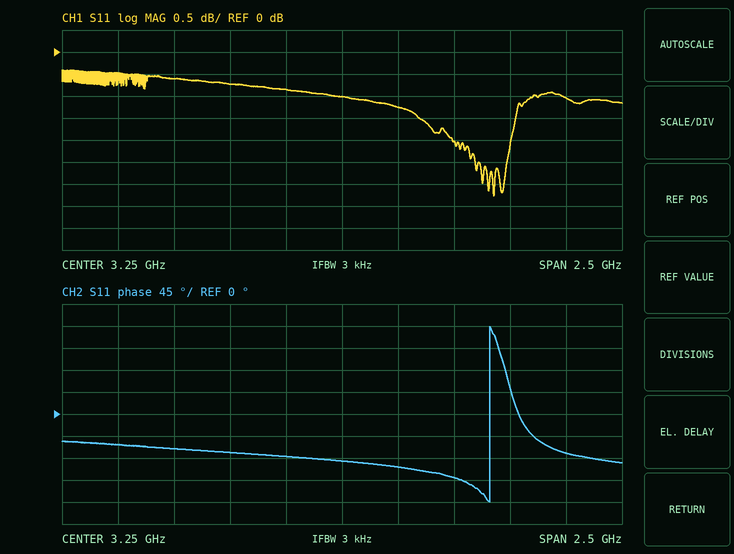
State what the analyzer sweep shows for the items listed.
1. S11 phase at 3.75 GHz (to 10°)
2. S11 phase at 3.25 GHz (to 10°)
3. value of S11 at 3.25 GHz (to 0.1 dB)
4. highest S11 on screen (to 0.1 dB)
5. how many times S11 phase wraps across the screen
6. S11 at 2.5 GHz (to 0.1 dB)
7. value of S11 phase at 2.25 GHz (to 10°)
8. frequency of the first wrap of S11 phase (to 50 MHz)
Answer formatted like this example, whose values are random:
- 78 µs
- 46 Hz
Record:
- -130°
- -100°
- -1.0 dB
- -0.4 dB
- 1
- -0.6 dB
- -60°
- 3.90 GHz
